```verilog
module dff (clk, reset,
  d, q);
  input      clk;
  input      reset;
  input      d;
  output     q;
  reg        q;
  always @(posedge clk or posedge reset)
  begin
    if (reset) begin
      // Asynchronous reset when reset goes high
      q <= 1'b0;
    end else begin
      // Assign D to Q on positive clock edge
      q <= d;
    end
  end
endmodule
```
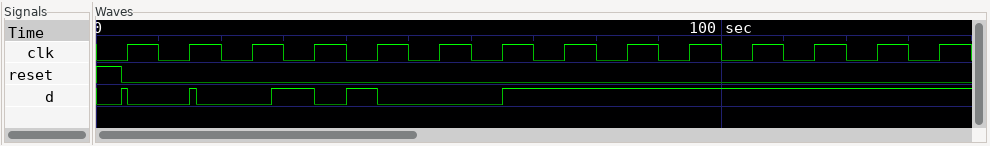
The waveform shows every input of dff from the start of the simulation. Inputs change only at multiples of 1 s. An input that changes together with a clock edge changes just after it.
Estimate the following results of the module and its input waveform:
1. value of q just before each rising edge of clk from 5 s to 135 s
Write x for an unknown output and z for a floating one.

0 1 0 0 1 1 0 0 1 1 1 1 1 1
